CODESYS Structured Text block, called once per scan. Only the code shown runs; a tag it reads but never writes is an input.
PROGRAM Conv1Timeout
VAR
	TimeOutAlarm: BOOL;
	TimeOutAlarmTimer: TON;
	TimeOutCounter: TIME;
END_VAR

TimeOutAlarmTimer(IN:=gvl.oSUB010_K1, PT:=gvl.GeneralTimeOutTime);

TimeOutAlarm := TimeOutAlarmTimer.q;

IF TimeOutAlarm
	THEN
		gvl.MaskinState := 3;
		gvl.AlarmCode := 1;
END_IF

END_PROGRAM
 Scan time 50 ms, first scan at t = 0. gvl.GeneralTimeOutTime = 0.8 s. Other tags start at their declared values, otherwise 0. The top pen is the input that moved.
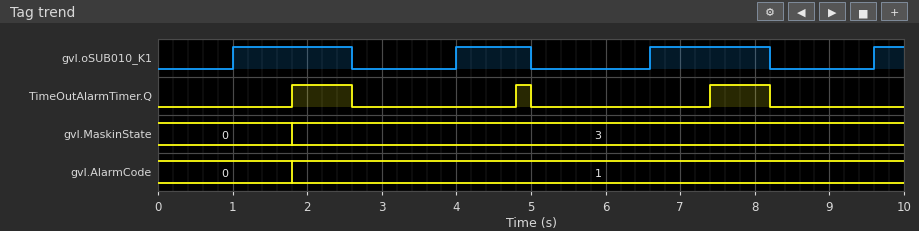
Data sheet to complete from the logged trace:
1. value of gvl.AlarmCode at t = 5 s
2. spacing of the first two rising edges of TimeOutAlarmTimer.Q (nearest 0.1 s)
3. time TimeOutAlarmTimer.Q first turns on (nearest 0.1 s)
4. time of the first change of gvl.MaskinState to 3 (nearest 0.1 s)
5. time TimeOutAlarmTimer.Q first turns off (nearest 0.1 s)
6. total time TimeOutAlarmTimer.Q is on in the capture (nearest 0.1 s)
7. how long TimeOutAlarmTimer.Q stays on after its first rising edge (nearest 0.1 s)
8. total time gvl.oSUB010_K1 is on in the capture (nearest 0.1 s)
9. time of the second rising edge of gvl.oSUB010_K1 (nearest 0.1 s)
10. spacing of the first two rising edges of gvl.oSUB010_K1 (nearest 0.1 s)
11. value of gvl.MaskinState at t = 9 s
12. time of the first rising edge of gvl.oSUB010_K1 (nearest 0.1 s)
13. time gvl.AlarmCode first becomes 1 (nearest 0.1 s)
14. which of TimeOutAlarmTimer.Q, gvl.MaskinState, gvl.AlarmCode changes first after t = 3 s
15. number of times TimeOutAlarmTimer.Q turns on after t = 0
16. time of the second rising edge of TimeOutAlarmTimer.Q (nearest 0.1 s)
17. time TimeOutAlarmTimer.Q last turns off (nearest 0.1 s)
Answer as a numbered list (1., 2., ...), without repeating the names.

1. 1
2. 3.0 s
3. 1.8 s
4. 1.8 s
5. 2.6 s
6. 1.8 s
7. 0.8 s
8. 4.6 s
9. 4.0 s
10. 3.0 s
11. 3
12. 1.0 s
13. 1.8 s
14. TimeOutAlarmTimer.Q
15. 3
16. 4.8 s
17. 8.2 s
